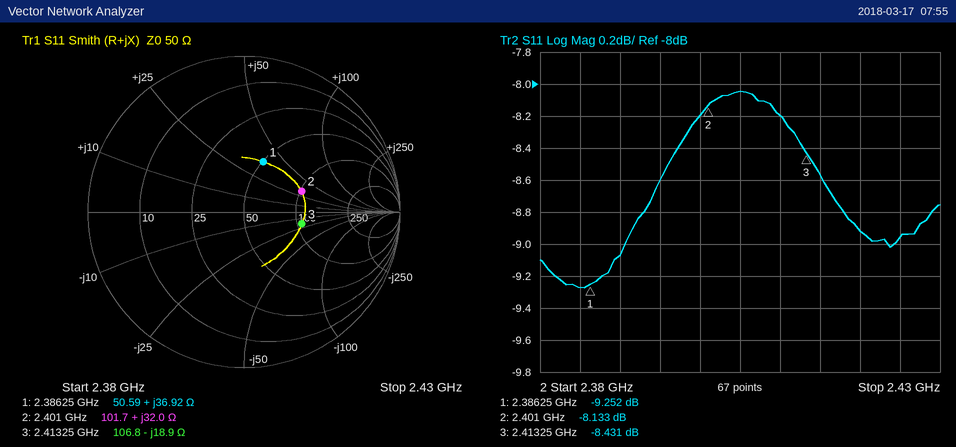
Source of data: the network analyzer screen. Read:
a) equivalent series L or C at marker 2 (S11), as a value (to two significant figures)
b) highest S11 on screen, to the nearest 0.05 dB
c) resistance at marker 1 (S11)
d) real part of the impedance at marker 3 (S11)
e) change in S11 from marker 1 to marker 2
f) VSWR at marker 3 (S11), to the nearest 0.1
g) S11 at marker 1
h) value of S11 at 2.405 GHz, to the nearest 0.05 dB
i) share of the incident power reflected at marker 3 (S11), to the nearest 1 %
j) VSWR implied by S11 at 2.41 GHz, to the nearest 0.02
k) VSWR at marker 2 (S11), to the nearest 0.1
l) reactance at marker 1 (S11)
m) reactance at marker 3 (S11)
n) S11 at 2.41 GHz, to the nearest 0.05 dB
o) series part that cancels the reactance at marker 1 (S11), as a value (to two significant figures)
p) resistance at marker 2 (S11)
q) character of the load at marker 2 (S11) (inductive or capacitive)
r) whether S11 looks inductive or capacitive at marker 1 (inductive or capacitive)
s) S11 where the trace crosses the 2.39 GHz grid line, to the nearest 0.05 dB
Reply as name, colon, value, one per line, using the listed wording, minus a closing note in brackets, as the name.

equivalent series L or C at marker 2 (S11), as a value: 2.1 nH
highest S11 on screen, to the nearest 0.05 dB: -8.05 dB
resistance at marker 1: 50.59 Ω
real part of the impedance at marker 3: 106.8 Ω
change in S11 from marker 1 to marker 2: 1.119 dB
VSWR at marker 3 (S11), to the nearest 0.1: 2.2
S11 at marker 1: -9.252 dB
value of S11 at 2.405 GHz, to the nearest 0.05 dB: -8.05 dB
share of the incident power reflected at marker 3 (S11), to the nearest 1 %: 14 %
VSWR implied by S11 at 2.41 GHz, to the nearest 0.02: 2.28
VSWR at marker 2 (S11), to the nearest 0.1: 2.3
reactance at marker 1: +36.92 Ω
reactance at marker 3: -18.9 Ω
S11 at 2.41 GHz, to the nearest 0.05 dB: -8.20 dB
series part that cancels the reactance at marker 1 (S11), as a value: 1.8 pF
resistance at marker 2: 101.7 Ω
character of the load at marker 2 (S11): inductive
whether S11 looks inductive or capacitive at marker 1: inductive
S11 where the trace crosses the 2.39 GHz grid line, to the nearest 0.05 dB: -9.05 dB
